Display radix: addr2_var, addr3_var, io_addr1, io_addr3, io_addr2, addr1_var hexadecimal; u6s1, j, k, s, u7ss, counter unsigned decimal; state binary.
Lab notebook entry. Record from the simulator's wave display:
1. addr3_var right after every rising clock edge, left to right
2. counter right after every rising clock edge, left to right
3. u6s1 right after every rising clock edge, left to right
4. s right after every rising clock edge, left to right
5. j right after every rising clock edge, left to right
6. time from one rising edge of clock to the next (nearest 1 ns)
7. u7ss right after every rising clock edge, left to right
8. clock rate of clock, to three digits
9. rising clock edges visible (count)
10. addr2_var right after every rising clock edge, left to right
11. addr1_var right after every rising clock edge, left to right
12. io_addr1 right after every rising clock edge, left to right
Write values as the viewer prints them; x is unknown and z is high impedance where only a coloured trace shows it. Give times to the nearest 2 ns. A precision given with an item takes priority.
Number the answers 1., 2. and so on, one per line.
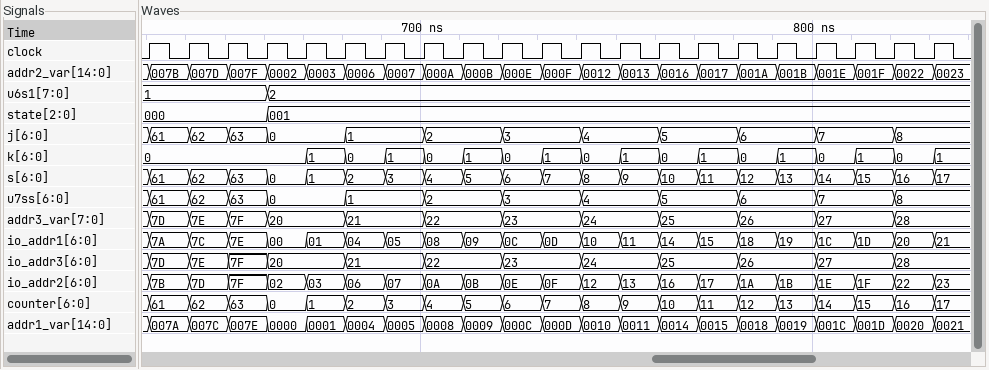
1. 7D, 7E, 7F, 20, 20, 21, 21, 22, 22, 23, 23, 24, 24, 25, 25, 26, 26, 27, 27, 28, 28
2. 61, 62, 63, 0, 1, 2, 3, 4, 5, 6, 7, 8, 9, 10, 11, 12, 13, 14, 15, 16, 17
3. 1, 1, 1, 2, 2, 2, 2, 2, 2, 2, 2, 2, 2, 2, 2, 2, 2, 2, 2, 2, 2
4. 61, 62, 63, 0, 1, 2, 3, 4, 5, 6, 7, 8, 9, 10, 11, 12, 13, 14, 15, 16, 17
5. 61, 62, 63, 0, 0, 1, 1, 2, 2, 3, 3, 4, 4, 5, 5, 6, 6, 7, 7, 8, 8
6. 10 ns
7. 61, 62, 63, 0, 0, 1, 1, 2, 2, 3, 3, 4, 4, 5, 5, 6, 6, 7, 7, 8, 8
8. 100 MHz
9. 21
10. 007B, 007D, 007F, 0002, 0003, 0006, 0007, 000A, 000B, 000E, 000F, 0012, 0013, 0016, 0017, 001A, 001B, 001E, 001F, 0022, 0023
11. 007A, 007C, 007E, 0000, 0001, 0004, 0005, 0008, 0009, 000C, 000D, 0010, 0011, 0014, 0015, 0018, 0019, 001C, 001D, 0020, 0021
12. 7A, 7C, 7E, 00, 01, 04, 05, 08, 09, 0C, 0D, 10, 11, 14, 15, 18, 19, 1C, 1D, 20, 21
